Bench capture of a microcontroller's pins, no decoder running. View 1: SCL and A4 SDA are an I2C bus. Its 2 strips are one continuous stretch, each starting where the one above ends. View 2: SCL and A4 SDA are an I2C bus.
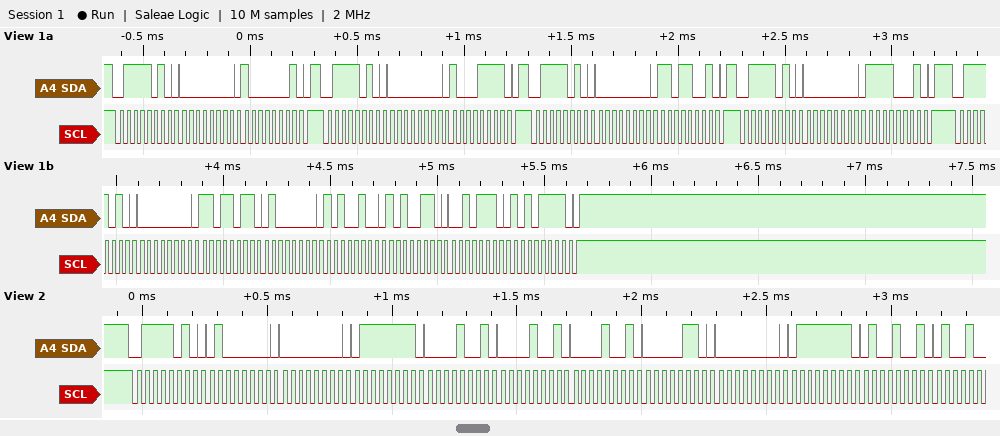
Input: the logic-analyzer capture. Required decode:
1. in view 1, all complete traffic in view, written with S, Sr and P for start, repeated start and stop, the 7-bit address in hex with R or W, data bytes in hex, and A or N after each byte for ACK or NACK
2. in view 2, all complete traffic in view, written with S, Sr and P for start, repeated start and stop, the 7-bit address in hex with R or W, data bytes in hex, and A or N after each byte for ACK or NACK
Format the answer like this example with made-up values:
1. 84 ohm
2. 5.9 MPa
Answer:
1. S 3DW A 00 A 81 A P S 3DW A 00 A 8F A P S 3DW A 00 A D9 A P S 3DW A 00 A F1 A P S 3DW A 00 A DB A 40 A A4 A A6 A 2E A AF A P
2. S 3DW A 40 A 00 A 7F A 09 A 09 A 09 A 06 A 00 A 7F A 49 A
